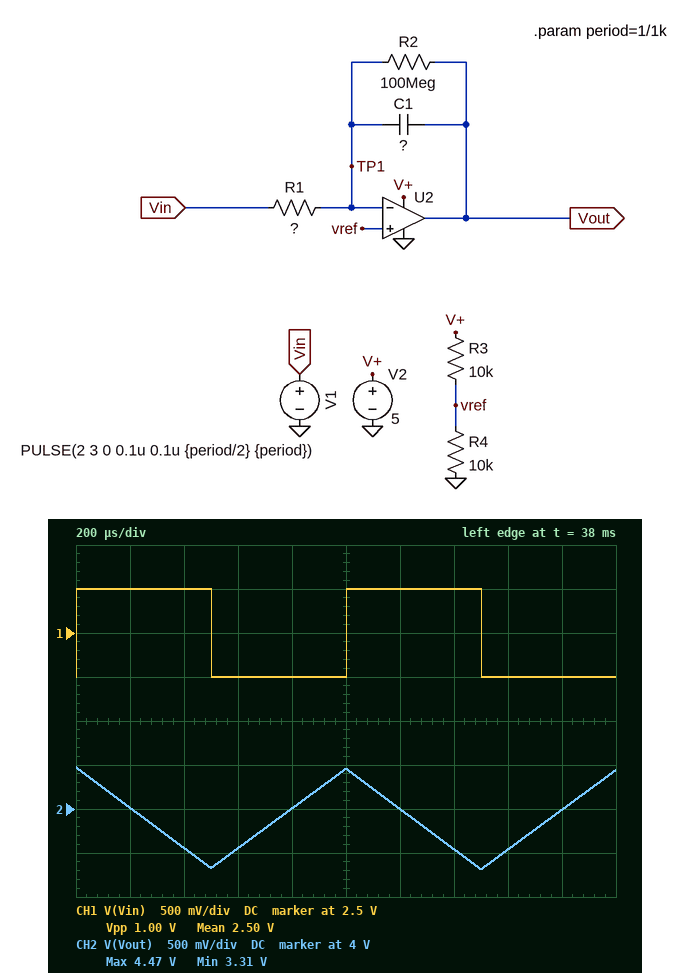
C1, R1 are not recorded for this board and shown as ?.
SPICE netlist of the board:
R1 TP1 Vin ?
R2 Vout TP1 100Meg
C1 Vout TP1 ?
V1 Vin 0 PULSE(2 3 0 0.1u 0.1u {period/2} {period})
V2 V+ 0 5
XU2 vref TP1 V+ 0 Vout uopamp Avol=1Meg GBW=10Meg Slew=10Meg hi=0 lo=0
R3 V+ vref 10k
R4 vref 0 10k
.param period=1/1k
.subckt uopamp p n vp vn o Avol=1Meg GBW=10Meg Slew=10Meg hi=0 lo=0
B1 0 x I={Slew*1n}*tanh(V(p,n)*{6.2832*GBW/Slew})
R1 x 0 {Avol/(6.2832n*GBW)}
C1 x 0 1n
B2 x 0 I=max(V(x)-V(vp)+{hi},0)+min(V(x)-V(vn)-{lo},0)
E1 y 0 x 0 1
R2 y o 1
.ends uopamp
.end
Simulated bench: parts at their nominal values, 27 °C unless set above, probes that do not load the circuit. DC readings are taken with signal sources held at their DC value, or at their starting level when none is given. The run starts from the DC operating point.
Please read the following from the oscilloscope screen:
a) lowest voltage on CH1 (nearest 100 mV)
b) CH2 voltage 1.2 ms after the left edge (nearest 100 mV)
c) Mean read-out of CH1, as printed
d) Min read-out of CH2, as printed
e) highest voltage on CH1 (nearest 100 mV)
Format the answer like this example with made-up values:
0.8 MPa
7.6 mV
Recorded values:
2.0 V
4.0 V
2.50 V
3.31 V
3.0 V
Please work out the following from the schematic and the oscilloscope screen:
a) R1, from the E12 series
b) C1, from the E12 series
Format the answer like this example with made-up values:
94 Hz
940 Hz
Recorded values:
220 kΩ
1 nF
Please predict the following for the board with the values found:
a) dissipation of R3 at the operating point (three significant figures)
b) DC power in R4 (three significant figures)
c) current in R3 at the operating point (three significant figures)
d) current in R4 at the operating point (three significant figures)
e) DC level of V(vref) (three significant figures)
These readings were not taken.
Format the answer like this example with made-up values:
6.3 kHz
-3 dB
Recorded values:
625 µW
625 µW
250 µA
250 µA
2.50 V
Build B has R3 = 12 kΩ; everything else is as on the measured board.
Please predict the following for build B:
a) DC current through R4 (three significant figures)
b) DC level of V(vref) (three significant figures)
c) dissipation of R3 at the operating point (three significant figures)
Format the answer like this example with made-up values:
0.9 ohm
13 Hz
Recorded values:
227 µA
2.27 V
620 µW
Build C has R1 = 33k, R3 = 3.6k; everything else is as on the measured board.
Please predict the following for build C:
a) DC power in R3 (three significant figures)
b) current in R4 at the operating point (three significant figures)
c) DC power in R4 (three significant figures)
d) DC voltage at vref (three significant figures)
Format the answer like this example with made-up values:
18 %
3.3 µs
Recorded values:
487 µW
368 µA
1.35 mW
3.68 V
